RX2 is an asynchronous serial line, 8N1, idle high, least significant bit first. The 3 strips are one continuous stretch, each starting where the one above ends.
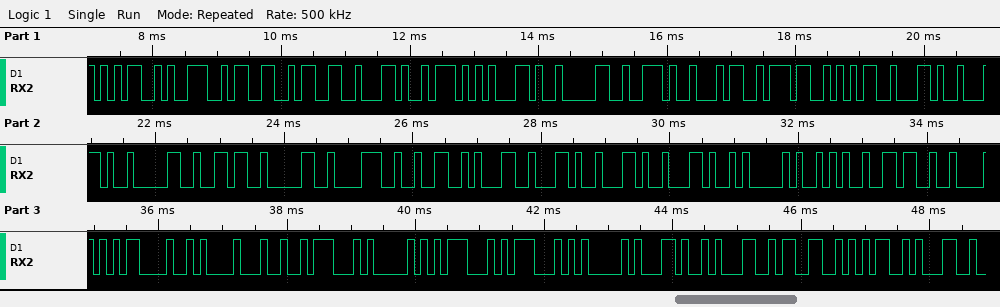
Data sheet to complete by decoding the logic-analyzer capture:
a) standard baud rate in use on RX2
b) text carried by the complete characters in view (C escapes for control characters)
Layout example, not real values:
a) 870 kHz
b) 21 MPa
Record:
a) 9600 baud
b) "5933,W,0.475,,060821,,,A*6B\r\n$GPGGA,1351"
